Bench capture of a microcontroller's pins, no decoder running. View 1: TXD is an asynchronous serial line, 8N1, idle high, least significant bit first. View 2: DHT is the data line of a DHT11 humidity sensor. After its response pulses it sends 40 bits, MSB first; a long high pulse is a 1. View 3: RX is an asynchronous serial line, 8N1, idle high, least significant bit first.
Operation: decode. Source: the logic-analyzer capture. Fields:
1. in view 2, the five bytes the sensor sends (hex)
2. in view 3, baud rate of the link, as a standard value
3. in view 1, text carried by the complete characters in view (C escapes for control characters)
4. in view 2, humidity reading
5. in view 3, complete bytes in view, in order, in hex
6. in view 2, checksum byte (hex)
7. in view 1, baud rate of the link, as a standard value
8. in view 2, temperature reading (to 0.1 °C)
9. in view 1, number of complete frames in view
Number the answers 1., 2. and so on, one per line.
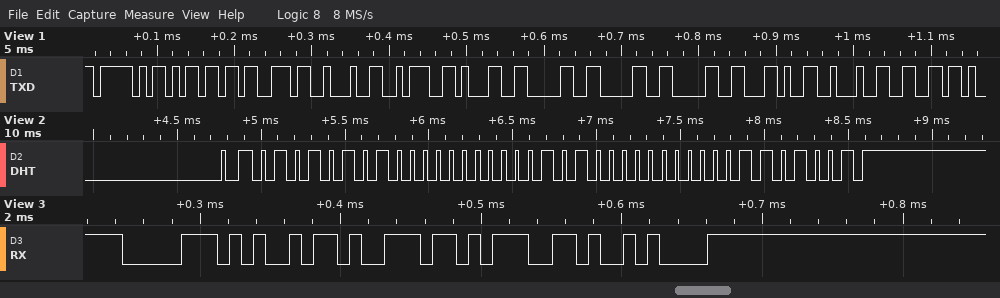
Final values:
1. 55 00 14 00 69
2. 115200 baud
3. "_ms\":1000,\"f"
4. 85 %
5. 70 69 6E 67 0A
6. 0x69
7. 115200 baud
8. 20.0 °C
9. 12
